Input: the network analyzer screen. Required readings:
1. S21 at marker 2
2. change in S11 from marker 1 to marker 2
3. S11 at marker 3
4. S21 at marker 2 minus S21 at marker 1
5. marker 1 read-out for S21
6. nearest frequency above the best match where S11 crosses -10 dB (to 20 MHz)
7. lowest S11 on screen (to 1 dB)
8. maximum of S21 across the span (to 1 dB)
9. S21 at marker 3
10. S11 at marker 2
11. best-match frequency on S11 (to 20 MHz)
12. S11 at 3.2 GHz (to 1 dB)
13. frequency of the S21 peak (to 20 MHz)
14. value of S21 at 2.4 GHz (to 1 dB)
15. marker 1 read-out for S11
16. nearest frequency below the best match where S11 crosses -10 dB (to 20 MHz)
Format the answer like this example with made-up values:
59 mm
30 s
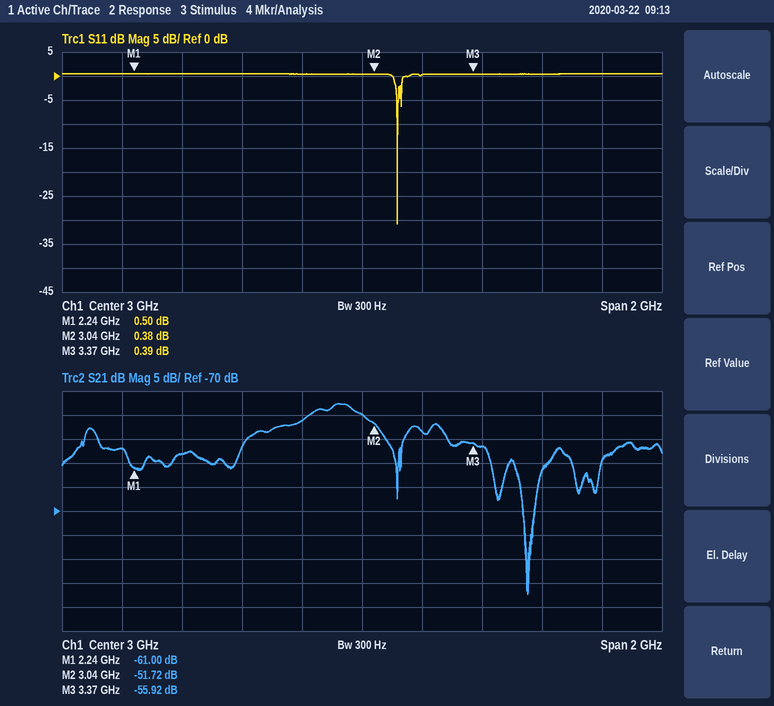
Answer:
-51.72 dB
-0.12 dB
0.39 dB
9.28 dB
-61.00 dB
3.12 GHz
-31 dB
-48 dB
-55.92 dB
0.38 dB
3.12 GHz
0 dB
2.92 GHz
-58 dB
0.50 dB
3.12 GHz
